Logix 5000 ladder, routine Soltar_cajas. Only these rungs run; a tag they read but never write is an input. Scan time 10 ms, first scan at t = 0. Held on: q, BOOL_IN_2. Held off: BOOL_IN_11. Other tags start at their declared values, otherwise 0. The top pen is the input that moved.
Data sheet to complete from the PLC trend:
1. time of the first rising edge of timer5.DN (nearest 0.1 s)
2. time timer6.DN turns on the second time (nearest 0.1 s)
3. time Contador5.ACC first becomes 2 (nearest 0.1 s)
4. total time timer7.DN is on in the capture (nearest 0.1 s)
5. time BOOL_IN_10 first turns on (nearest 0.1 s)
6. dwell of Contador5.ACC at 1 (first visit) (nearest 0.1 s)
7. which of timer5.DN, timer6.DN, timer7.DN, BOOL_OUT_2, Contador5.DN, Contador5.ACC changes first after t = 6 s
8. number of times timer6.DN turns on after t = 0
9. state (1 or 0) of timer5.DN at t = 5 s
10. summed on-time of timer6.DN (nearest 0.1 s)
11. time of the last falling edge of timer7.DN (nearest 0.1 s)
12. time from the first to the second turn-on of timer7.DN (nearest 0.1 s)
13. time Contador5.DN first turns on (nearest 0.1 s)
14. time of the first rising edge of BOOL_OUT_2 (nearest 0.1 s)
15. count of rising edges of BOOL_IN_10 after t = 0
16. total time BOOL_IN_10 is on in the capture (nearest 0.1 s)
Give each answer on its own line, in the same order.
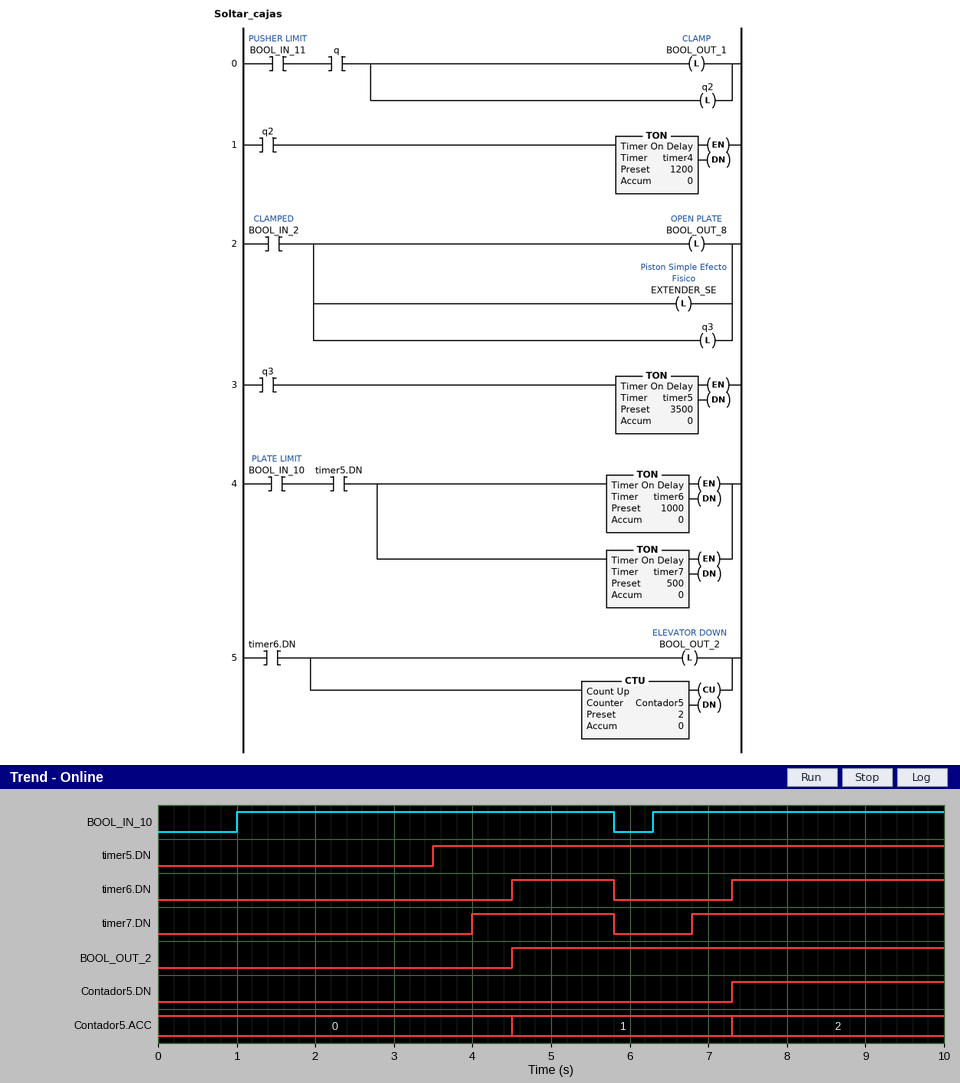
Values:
3.5 s
7.3 s
7.3 s
5.0 s
1.0 s
2.8 s
timer7.DN
2
1
4.0 s
5.8 s
2.8 s
7.3 s
4.5 s
2
8.5 s
